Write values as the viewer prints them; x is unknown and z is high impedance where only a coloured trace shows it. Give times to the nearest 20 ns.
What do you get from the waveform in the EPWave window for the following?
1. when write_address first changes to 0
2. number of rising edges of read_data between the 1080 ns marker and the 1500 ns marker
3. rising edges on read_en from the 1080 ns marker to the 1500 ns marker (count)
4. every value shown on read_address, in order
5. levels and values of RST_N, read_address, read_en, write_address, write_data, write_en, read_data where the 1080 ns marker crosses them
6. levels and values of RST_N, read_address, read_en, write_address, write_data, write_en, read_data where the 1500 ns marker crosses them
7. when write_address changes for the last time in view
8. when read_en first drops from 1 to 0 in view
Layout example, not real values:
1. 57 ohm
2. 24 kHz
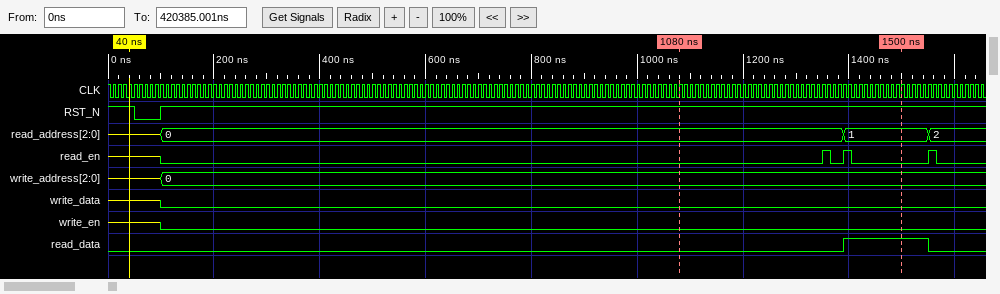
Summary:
1. 100 ns
2. 1
3. 2
4. z, 0, 1, 2
5. RST_N=1, read_address=0, read_en=0, write_address=0, write_data=0, write_en=0, read_data=0
6. RST_N=1, read_address=1, read_en=0, write_address=0, write_data=0, write_en=0, read_data=1
7. 100 ns
8. 1360 ns
